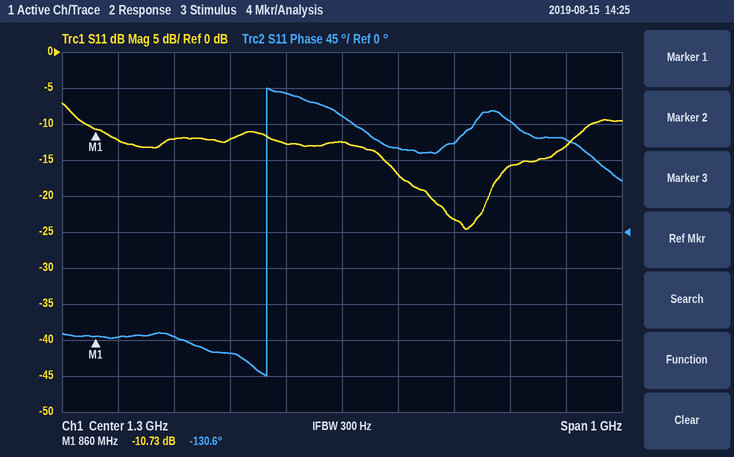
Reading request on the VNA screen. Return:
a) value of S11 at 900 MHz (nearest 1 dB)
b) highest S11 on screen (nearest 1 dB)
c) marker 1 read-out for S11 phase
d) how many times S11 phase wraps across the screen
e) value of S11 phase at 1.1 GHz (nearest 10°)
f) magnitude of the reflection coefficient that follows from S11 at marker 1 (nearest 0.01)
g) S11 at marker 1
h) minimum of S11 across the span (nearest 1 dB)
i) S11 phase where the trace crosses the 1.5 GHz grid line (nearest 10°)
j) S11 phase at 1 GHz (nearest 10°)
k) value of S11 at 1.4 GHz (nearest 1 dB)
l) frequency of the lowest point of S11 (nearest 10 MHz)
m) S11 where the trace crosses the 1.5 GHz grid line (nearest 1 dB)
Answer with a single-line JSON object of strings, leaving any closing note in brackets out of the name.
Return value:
{"value of S11 at 900 MHz": "-12 dB", "highest S11 on screen": "-7 dB", "marker 1 read-out for S11 phase": "-130.6°", "how many times S11 phase wraps across the screen": "1", "value of S11 phase at 1.1 GHz": "-150°", "magnitude of the reflection coefficient that follows from S11 at marker 1": "0.29", "S11 at marker 1": "-10.73 dB", "minimum of S11 across the span": "-25 dB", "S11 phase where the trace crosses the 1.5 GHz grid line": "110°", "S11 phase at 1 GHz": "-130°", "value of S11 at 1.4 GHz": "-17 dB", "frequency of the lowest point of S11": "1.52 GHz", "S11 where the trace crosses the 1.5 GHz grid line": "-23 dB"}
